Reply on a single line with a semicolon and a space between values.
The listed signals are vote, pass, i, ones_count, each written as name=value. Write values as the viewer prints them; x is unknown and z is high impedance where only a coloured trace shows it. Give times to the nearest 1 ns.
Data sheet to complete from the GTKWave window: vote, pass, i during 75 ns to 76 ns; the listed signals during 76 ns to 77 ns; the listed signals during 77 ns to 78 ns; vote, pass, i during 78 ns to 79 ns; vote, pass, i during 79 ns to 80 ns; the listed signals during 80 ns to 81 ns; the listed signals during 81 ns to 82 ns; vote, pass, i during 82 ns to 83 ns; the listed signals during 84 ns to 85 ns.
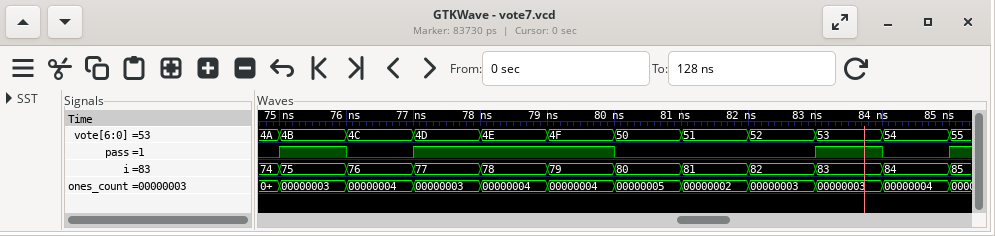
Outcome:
vote=4B, pass=1, i=75; vote=4C, pass=0, i=76, ones_count=00000004; vote=4D, pass=1, i=77, ones_count=00000003; vote=4E, pass=1, i=78; vote=4F, pass=1, i=79; vote=50, pass=0, i=80, ones_count=00000005; vote=51, pass=0, i=81, ones_count=00000002; vote=52, pass=0, i=82; vote=54, pass=0, i=84, ones_count=00000004
